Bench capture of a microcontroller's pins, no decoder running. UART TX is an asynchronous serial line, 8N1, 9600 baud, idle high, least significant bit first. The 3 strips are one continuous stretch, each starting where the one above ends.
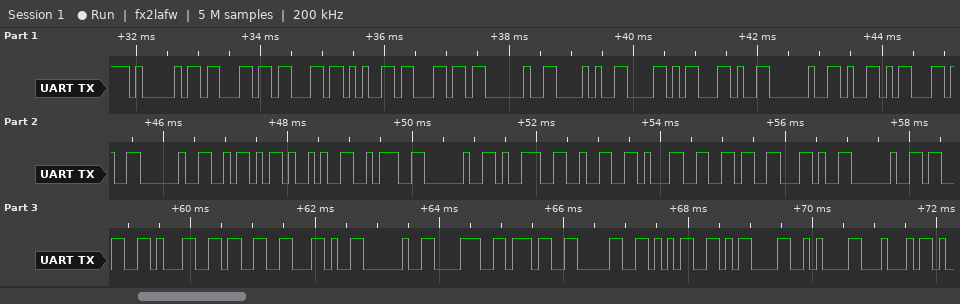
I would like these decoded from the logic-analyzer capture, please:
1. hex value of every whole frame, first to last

0x41 0x63 0x63 0x65 0x6C 0x20 0x28 0x58 0x2C 0x20 0x59 0x2C 0x20 0x5A 0x29 0x3A 0x20 0x39 0x32 0x31 0x36 0x2C 0x20 0x33 0x31 0x33 0x2C 0x20 0x38 0x37 0x30 0x35 0x0D 0x0A 0x44
